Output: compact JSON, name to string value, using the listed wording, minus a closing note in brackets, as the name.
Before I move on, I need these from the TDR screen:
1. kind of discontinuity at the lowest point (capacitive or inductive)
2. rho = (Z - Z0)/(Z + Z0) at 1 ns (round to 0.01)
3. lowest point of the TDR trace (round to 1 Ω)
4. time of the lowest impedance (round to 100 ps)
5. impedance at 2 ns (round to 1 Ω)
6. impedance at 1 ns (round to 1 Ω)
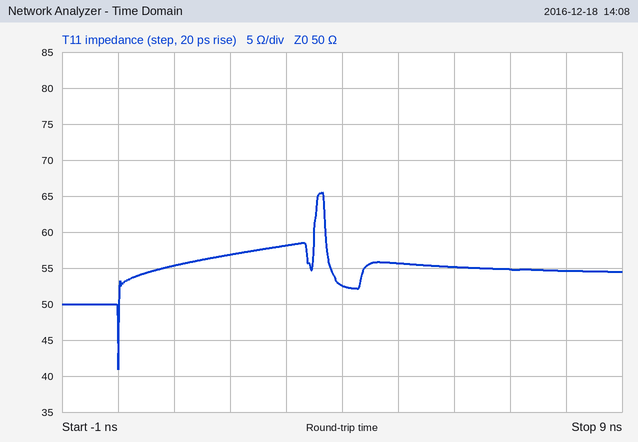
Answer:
{"kind of discontinuity at the lowest point": "capacitive", "rho = (Z - Z0)/(Z + Z0) at 1 ns": "+0.05", "lowest point of the TDR trace": "41 Ω", "time of the lowest impedance": "0.0 ns", "impedance at 2 ns": "57 Ω", "impedance at 1 ns": "55 Ω"}
